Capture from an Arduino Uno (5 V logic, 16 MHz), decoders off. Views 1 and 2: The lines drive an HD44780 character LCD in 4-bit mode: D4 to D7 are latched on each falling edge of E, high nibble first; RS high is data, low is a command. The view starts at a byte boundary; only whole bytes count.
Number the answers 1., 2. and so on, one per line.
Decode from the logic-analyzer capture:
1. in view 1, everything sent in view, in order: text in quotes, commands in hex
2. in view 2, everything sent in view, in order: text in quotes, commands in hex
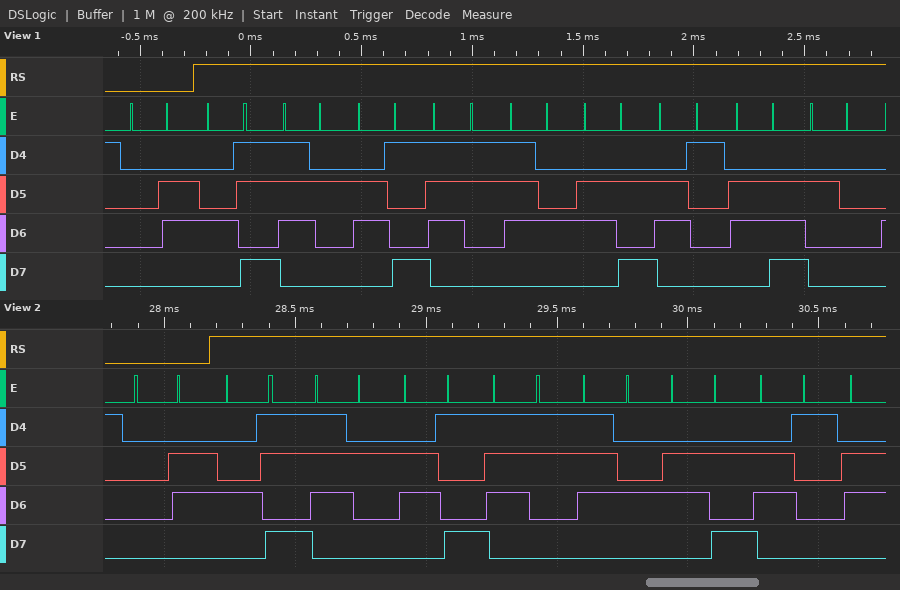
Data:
1. 0x06 "Kristjan "
2. 0x06 "Kristja"
